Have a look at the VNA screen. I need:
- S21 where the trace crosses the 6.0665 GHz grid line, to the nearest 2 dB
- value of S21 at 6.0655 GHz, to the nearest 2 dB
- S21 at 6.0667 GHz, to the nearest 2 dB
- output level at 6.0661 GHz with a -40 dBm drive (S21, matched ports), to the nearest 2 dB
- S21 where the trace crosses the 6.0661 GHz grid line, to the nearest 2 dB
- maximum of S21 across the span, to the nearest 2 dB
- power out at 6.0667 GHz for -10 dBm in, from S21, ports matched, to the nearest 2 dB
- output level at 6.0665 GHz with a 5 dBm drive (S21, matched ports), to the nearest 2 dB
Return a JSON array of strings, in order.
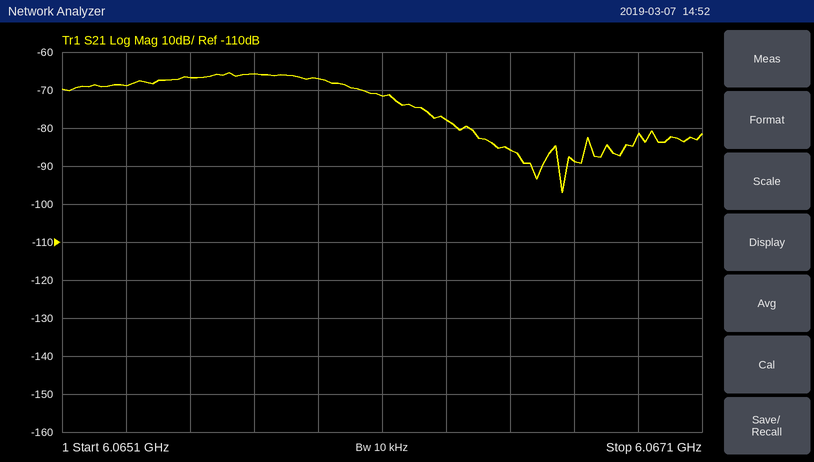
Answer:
["-86 dB", "-66 dB", "-88 dB", "-112 dBm", "-72 dB", "-66 dB", "-98 dBm", "-80 dBm"]
